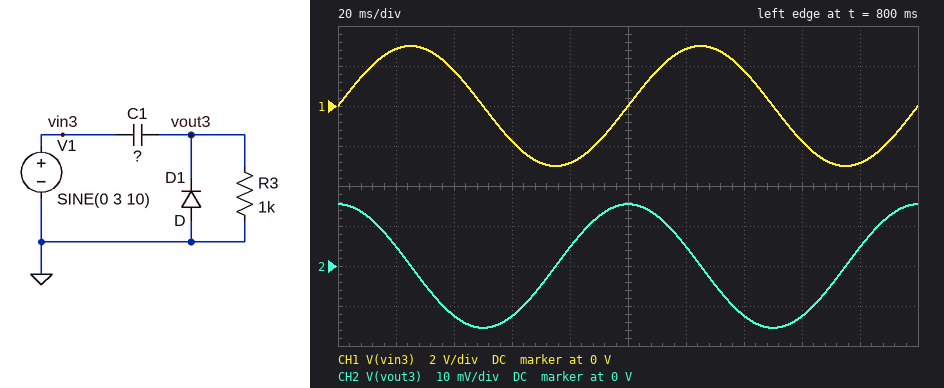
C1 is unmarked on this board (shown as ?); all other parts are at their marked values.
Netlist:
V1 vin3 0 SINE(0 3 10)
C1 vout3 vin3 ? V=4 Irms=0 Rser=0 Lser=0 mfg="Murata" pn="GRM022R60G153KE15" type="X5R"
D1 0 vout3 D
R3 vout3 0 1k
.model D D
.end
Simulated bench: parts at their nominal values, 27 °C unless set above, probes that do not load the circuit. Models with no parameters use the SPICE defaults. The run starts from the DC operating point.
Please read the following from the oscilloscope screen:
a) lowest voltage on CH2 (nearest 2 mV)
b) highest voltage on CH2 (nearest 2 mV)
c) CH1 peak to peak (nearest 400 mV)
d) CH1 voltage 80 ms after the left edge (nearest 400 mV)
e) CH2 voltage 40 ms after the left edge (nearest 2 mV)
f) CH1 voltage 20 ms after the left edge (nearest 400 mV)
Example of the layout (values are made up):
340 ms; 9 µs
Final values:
-16 mV; 16 mV; 6.0 V; -2.8 V; -12 mV; 2.8 V
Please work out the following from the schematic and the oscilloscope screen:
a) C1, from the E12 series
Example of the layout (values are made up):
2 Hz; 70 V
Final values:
82 nF
